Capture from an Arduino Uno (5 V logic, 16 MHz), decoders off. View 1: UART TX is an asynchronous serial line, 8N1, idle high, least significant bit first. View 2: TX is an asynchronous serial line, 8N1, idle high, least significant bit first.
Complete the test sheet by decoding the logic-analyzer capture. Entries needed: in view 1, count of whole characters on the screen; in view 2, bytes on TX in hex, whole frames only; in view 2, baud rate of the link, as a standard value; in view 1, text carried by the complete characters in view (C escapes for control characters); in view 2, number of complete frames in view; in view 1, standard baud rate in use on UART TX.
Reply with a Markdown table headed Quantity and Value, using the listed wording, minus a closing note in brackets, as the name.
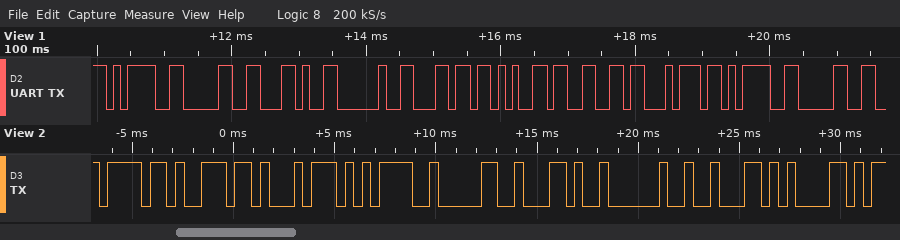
| Quantity | Value |
|---|---|
| in view 1, count of whole characters on the screen | 10 |
| in view 2, bytes on TX in hex, whole frames only | 0x6F 0x6E 0x74 0x3D 0x30 0x2C 0x20 0x62 0x61 |
| in view 2, baud rate of the link, as a standard value | 2400 baud |
| in view 1, text carried by the complete characters in view | "=0, left=0" |
| in view 2, number of complete frames in view | 9 |
| in view 1, standard baud rate in use on UART TX | 9600 baud |
